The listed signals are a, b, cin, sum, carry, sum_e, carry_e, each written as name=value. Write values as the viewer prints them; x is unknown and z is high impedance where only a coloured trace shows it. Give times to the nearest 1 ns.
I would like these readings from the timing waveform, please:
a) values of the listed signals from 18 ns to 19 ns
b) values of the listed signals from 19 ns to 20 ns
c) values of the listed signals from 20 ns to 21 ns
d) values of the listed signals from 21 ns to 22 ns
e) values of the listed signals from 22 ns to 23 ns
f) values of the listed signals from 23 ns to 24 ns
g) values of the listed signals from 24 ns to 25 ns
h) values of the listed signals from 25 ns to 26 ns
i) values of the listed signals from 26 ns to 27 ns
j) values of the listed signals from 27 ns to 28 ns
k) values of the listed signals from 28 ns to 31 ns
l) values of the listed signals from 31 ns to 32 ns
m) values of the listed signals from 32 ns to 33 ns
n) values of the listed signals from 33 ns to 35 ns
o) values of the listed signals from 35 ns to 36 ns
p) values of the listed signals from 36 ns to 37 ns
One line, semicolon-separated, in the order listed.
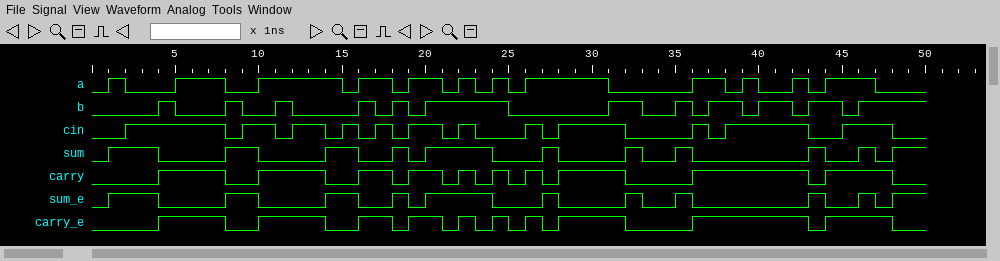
a=0, b=1, cin=0, sum=1, carry=0, sum_e=1, carry_e=0; a=1, b=0, cin=1, sum=0, carry=1, sum_e=0, carry_e=1; a=1, b=1, cin=1, sum=1, carry=1, sum_e=1, carry_e=1; a=0, b=1, cin=0, sum=1, carry=0, sum_e=1, carry_e=0; a=1, b=1, cin=1, sum=1, carry=1, sum_e=1, carry_e=1; a=0, b=1, cin=0, sum=1, carry=0, sum_e=1, carry_e=0; a=1, b=1, cin=0, sum=0, carry=1, sum_e=0, carry_e=1; a=0, b=0, cin=0, sum=0, carry=0, sum_e=0, carry_e=0; a=1, b=0, cin=1, sum=0, carry=1, sum_e=0, carry_e=1; a=1, b=0, cin=0, sum=1, carry=0, sum_e=1, carry_e=0; a=1, b=0, cin=1, sum=0, carry=1, sum_e=0, carry_e=1; a=0, b=1, cin=1, sum=0, carry=1, sum_e=0, carry_e=1; a=0, b=1, cin=0, sum=1, carry=0, sum_e=1, carry_e=0; a=0, b=0, cin=0, sum=0, carry=0, sum_e=0, carry_e=0; a=0, b=1, cin=0, sum=1, carry=0, sum_e=1, carry_e=0; a=1, b=0, cin=1, sum=0, carry=1, sum_e=0, carry_e=1
